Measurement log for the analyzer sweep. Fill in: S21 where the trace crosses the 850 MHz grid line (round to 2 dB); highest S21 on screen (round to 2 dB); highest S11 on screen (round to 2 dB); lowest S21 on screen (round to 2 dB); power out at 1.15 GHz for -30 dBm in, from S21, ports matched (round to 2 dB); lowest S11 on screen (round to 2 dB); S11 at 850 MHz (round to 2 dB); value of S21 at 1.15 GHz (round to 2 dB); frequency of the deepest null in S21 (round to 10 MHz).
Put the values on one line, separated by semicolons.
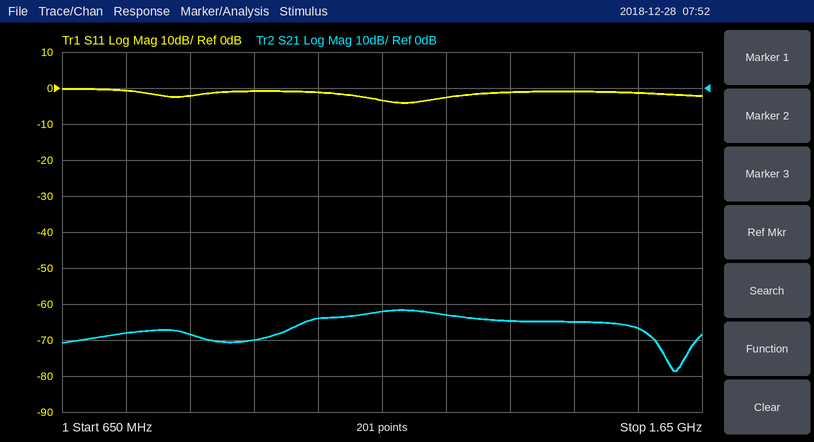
-68 dB; -62 dB; 0 dB; -78 dB; -92 dBm; -4 dB; -2 dB; -62 dB; 1.61 GHz
